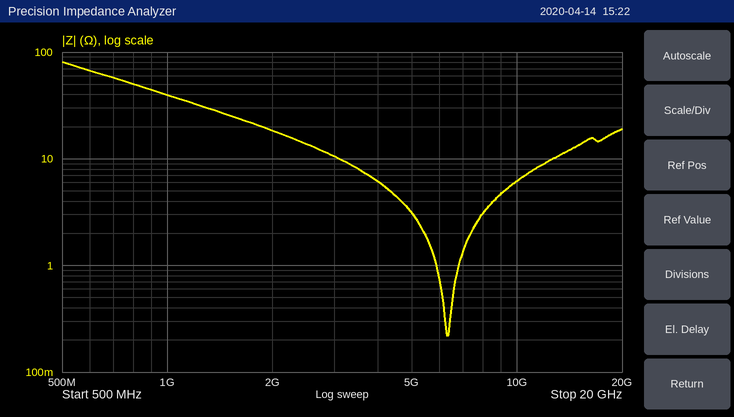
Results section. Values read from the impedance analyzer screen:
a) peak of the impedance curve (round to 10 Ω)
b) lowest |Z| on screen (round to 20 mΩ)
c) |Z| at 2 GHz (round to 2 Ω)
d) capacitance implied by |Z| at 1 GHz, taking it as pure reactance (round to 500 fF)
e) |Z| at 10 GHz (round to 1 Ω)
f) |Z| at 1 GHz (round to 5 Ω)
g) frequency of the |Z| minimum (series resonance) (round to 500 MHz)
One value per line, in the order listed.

80 Ω
220 mΩ
18 Ω
4.0 pF
6 Ω
40 Ω
6.5 GHz
